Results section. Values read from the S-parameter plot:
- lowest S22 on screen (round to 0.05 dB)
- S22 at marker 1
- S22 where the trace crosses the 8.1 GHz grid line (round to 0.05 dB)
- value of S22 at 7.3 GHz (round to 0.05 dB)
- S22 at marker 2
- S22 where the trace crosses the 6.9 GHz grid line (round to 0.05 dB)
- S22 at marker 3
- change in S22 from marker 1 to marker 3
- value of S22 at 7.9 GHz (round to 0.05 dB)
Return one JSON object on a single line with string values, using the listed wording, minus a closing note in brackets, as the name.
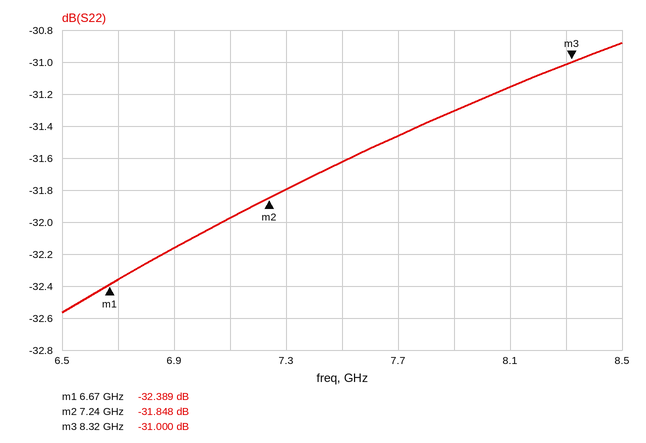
{"lowest S22 on screen": "-32.55 dB", "S22 at marker 1": "-32.389 dB", "S22 where the trace crosses the 8.1 GHz grid line": "-31.15 dB", "value of S22 at 7.3 GHz": "-31.80 dB", "S22 at marker 2": "-31.848 dB", "S22 where the trace crosses the 6.9 GHz grid line": "-32.15 dB", "S22 at marker 3": "-31.000 dB", "change in S22 from marker 1 to marker 3": "1.389 dB", "value of S22 at 7.9 GHz": "-31.30 dB"}
